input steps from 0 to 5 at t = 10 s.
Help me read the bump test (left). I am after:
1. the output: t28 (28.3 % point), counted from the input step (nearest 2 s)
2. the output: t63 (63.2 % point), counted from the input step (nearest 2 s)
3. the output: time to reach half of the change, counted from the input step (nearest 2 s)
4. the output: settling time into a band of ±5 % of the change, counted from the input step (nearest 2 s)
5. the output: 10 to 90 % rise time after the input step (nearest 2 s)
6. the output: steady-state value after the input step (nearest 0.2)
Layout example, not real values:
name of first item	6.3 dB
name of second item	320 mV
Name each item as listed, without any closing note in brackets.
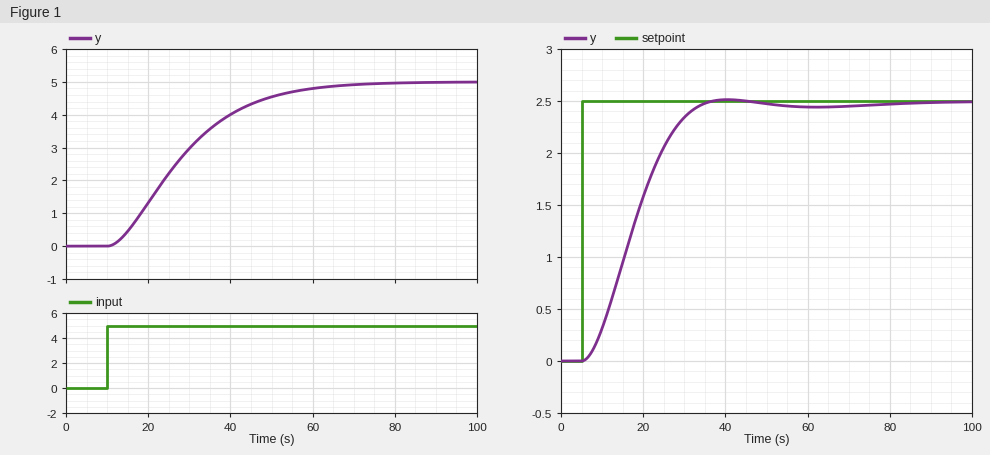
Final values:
the output: t28 (28.3 % point), counted from the input step	10 s
the output: t63 (63.2 % point), counted from the input step	22 s
the output: time to reach half of the change, counted from the input step	16 s
the output: settling time into a band of ±5 % of the change, counted from the input step	48 s
the output: 10 to 90 % rise time after the input step	34 s
the output: steady-state value after the input step	5.0
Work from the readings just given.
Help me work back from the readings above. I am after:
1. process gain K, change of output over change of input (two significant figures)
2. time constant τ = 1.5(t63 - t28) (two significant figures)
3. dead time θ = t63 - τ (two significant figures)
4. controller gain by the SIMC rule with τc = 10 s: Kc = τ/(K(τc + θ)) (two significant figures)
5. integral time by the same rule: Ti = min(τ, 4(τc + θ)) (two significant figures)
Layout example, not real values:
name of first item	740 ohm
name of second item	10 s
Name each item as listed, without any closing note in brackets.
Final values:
process gain K, change of output over change of input	1.0
time constant τ = 1.5(t63 - t28)	18 s
dead time θ = t63 - τ	4.0 s
controller gain by the SIMC rule with τc = 10 s: Kc = τ/(K(τc + θ))	1.3
integral time by the same rule: Ti = min(τ, 4(τc + θ))	18 s
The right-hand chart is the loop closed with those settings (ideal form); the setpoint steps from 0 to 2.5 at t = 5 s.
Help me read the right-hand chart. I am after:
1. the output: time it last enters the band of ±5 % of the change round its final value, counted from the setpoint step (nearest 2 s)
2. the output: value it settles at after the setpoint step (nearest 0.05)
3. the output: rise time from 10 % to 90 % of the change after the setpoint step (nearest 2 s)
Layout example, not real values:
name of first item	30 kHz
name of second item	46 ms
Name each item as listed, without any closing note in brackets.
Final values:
the output: time it last enters the band of ±5 % of the change round its final value, counted from the setpoint step	26 s
the output: value it settles at after the setpoint step	2.50
the output: rise time from 10 % to 90 % of the change after the setpoint step	18 s
